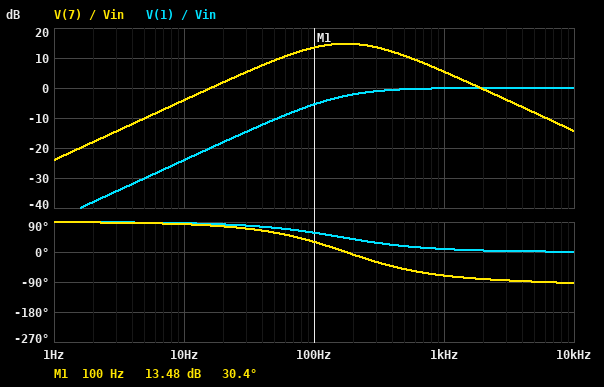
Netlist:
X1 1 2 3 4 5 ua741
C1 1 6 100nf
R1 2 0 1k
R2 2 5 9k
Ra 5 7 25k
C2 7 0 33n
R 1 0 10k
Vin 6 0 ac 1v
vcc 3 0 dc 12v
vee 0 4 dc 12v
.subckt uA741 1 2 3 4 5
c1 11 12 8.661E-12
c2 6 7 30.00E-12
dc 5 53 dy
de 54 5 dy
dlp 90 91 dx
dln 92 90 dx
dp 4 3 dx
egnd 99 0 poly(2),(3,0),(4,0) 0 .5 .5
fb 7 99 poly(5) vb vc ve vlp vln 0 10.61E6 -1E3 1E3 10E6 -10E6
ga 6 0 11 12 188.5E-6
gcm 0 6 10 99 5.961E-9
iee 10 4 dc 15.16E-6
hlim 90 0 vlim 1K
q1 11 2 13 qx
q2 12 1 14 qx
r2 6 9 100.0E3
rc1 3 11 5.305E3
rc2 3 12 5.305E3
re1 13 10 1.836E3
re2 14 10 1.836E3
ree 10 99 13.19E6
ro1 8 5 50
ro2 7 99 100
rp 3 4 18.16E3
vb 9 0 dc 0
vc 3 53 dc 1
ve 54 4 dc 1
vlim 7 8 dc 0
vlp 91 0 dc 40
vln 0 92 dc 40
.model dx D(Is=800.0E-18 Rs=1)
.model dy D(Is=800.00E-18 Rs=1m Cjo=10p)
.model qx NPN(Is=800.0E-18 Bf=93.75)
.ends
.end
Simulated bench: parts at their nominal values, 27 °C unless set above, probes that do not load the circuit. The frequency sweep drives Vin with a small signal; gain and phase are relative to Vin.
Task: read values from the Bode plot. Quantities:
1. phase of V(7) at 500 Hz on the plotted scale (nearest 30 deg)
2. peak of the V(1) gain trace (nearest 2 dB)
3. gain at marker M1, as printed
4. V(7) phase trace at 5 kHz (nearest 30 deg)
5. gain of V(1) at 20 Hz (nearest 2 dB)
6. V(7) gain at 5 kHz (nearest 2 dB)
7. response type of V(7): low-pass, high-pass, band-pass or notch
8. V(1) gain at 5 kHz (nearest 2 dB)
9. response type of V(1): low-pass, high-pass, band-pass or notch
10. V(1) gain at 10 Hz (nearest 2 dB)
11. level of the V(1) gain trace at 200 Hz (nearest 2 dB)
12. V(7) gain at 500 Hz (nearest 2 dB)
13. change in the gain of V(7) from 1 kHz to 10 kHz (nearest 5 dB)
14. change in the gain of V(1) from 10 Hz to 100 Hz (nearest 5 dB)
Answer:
-60 deg
0 dB
13.48 dB
-90 deg
-18 dB
-8 dB
band-pass
0 dB
high-pass
-24 dB
-2 dB
10 dB
-20 dB
20 dB
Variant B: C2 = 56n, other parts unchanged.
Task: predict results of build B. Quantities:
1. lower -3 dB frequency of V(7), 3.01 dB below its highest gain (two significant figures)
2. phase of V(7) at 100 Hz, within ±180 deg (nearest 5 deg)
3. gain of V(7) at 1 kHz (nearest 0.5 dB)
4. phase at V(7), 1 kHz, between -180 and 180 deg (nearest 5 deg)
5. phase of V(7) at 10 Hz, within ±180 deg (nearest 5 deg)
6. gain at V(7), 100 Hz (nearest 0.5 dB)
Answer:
55 Hz
15 deg
1.0 dB
-75 deg
80 deg
12.0 dB
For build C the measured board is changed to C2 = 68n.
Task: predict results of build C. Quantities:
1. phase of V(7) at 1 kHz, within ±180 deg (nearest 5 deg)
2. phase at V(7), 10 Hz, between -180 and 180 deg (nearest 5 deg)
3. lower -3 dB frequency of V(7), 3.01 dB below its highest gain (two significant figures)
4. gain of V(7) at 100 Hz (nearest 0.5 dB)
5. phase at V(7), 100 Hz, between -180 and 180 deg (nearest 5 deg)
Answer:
-75 deg
80 deg
49 Hz
11.0 dB
10 deg
